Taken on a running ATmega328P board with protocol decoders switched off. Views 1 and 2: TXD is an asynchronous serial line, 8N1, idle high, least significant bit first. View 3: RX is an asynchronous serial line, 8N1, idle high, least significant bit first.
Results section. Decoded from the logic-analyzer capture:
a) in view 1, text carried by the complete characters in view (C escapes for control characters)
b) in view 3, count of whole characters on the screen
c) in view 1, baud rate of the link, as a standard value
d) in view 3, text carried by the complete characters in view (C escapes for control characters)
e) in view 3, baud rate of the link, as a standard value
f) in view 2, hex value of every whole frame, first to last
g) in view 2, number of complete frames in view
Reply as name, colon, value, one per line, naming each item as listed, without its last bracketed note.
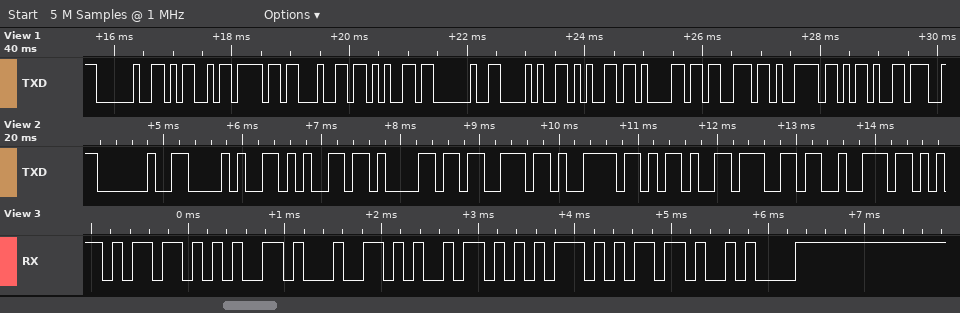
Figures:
in view 1, text carried by the complete characters in view: " Mode (easy-"
in view 3, count of whole characters on the screen: 7
in view 1, baud rate of the link, as a standard value: 9600 baud
in view 3, text carried by the complete characters in view: "medium\n"
in view 3, baud rate of the link, as a standard value: 9600 baud
in view 2, hex value of every whole frame, first to last: 0x20 0x28 0x65 0x61 0x73 0x79 0x2D 0x67 0x72
in view 2, number of complete frames in view: 9
